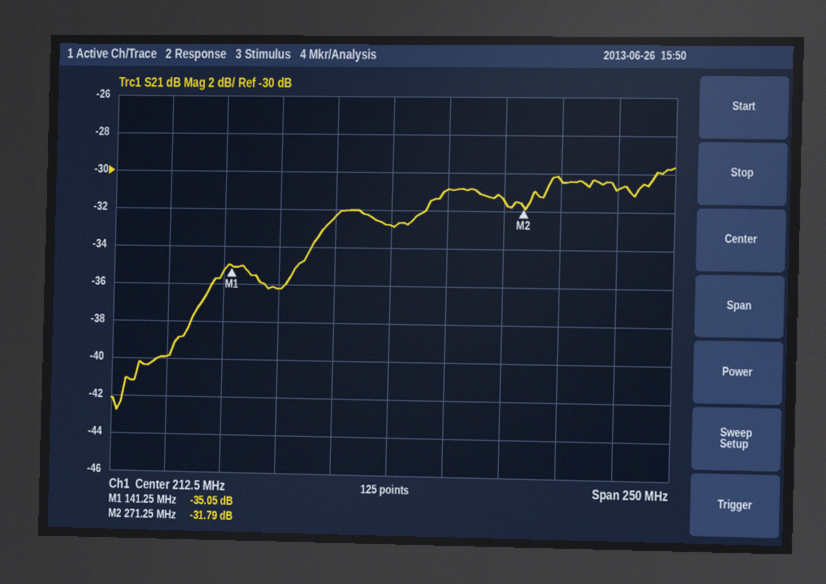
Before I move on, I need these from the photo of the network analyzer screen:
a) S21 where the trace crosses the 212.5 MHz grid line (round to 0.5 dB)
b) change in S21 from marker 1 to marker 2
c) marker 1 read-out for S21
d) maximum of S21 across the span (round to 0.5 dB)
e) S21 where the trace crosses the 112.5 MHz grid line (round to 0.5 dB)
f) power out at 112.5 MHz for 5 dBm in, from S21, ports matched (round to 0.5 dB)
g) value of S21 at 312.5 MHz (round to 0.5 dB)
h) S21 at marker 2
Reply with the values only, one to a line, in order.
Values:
-33.0 dB
3.26 dB
-35.05 dB
-29.5 dB
-40.0 dB
-35.0 dBm
-31.0 dB
-31.79 dB
